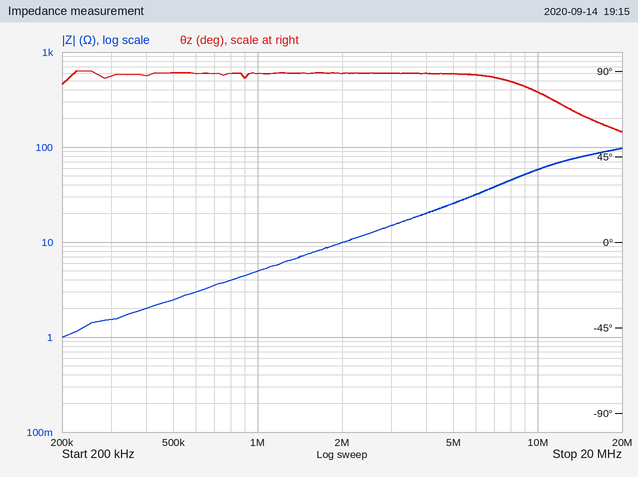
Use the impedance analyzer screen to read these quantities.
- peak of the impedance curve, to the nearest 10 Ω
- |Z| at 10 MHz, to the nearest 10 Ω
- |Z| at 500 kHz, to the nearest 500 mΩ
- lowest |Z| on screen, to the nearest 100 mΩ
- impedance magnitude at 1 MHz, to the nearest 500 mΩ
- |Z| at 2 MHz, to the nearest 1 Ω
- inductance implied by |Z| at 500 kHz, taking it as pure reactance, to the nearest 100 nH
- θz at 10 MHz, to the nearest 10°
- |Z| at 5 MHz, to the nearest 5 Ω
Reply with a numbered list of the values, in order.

1. 100 Ω
2. 60 Ω
3. 2.5 Ω
4. 1.0 Ω
5. 5.0 Ω
6. 10 Ω
7. 800 nH
8. 80°
9. 25 Ω
